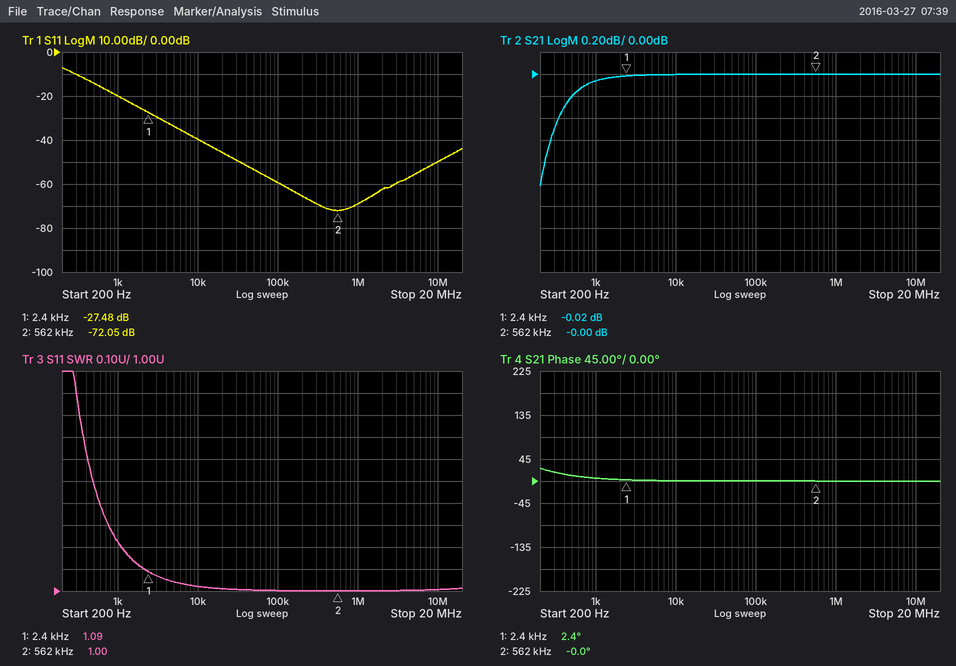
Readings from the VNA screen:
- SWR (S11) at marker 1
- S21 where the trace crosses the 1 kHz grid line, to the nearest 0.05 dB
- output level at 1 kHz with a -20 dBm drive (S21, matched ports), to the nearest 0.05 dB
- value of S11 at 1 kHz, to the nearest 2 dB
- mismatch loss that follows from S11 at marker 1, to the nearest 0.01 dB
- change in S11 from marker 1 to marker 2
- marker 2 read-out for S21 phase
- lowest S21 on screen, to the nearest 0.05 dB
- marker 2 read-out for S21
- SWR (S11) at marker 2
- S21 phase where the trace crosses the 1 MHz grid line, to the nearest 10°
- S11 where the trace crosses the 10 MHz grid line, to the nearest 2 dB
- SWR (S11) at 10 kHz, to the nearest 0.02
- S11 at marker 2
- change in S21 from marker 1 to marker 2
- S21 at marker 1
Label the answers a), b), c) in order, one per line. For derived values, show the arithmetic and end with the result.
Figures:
a) 1.09
b) -0.05 dB
c) -20 dBm + (-0.05 dB) = -20.05 dBm
d) -20 dB
e) −10 log10(1 − 10^(-27.48/10)) ≈ 0.01 dB
f) -72.05 − (-27.48) = -44.57 dB
g) -0.0°
h) -1.00 dB
i) -0.00 dB
j) 1.00
k) 0°
l) -50 dB
m) 1.02
n) -72.05 dB
o) -0 − (-0.02) = 0.02 dB
p) -0.02 dB
